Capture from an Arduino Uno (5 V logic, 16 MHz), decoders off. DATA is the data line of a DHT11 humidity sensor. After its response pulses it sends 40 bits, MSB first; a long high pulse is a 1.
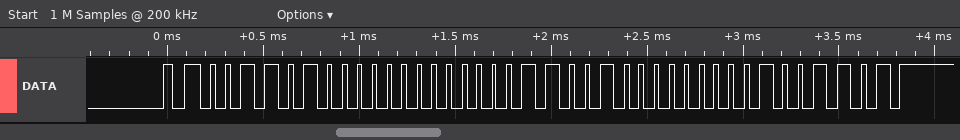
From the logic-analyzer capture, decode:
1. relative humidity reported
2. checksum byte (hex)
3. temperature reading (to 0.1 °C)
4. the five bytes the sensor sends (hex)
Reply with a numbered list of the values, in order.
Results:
1. 52 %
2. 0x4D
3. 25.0 °C
4. 34 00 19 00 4D
